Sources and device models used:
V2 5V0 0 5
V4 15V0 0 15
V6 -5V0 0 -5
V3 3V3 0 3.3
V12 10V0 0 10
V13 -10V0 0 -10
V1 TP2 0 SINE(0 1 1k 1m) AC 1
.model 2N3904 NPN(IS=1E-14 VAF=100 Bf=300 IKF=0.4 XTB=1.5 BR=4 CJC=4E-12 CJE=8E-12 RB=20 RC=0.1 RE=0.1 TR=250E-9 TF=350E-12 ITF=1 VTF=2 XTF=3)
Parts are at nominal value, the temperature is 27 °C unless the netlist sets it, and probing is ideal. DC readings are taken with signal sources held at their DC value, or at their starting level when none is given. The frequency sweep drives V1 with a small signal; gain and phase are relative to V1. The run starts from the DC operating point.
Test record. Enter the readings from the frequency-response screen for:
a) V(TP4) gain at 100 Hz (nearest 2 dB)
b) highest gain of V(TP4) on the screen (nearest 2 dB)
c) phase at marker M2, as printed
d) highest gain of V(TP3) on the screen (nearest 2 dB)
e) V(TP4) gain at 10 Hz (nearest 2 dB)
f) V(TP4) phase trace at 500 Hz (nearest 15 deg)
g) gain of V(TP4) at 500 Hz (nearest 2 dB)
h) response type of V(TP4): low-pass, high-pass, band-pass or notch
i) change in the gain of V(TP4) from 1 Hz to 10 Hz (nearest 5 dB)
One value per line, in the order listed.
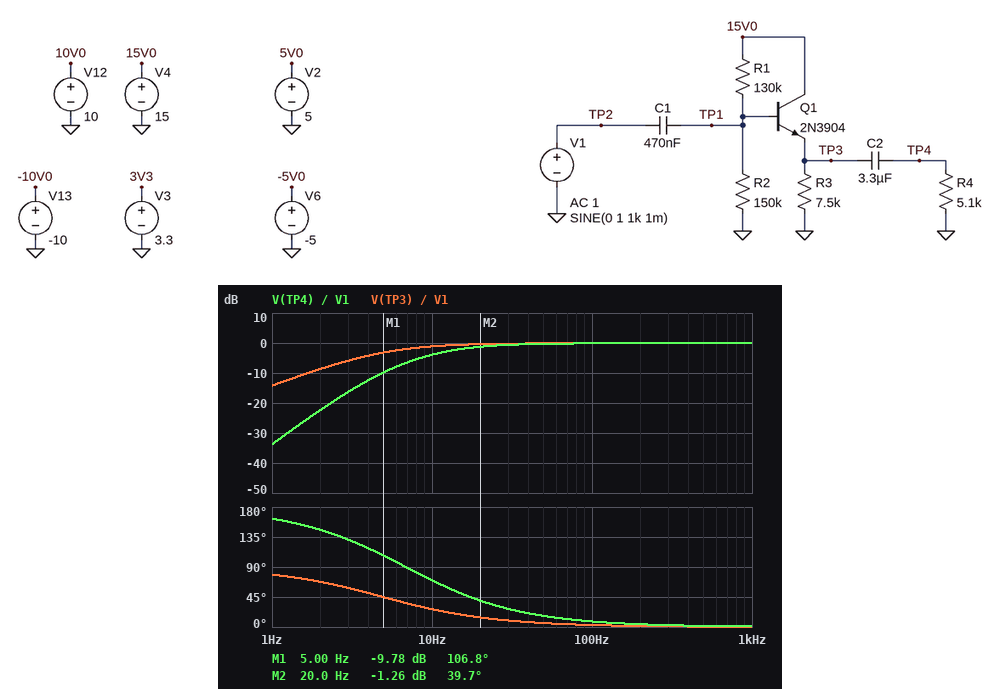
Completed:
0 dB
0 dB
39.7 deg
0 dB
-4 dB
0 deg
0 dB
high-pass
30 dB
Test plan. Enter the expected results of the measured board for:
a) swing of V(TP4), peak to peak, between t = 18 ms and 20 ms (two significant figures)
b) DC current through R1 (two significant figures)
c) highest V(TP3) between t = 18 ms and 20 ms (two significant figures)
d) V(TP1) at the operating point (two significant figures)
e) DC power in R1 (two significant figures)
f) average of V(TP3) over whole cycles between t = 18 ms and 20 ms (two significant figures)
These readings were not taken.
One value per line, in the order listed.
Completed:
2.0 V
55 µA
8.2 V
7.8 V
400 µW
7.2 V
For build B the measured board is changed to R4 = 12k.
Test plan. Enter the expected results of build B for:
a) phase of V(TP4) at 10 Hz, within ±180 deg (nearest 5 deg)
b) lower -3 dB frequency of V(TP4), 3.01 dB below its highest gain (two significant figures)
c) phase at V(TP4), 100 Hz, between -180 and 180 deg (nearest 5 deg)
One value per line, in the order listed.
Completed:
50 deg
7.1 Hz
5 deg
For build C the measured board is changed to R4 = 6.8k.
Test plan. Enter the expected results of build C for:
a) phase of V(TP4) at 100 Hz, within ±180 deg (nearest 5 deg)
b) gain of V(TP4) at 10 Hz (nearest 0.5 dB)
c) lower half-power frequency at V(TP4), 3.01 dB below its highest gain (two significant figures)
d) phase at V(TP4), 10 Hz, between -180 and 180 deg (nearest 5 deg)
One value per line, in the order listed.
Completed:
5 deg
-3.0 dB
9.6 Hz
60 deg
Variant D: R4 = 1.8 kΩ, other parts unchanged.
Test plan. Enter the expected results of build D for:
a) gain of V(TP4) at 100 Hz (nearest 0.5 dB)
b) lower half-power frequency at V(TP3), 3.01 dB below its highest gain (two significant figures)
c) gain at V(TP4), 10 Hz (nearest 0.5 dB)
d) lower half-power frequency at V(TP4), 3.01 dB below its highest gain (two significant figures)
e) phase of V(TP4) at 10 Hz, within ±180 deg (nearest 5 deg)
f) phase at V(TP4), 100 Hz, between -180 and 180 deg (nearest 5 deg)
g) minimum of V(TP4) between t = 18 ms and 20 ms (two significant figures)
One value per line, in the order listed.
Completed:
-0.5 dB
5.0 Hz
-10.5 dB
28 Hz
95 deg
20 deg
-970 mV
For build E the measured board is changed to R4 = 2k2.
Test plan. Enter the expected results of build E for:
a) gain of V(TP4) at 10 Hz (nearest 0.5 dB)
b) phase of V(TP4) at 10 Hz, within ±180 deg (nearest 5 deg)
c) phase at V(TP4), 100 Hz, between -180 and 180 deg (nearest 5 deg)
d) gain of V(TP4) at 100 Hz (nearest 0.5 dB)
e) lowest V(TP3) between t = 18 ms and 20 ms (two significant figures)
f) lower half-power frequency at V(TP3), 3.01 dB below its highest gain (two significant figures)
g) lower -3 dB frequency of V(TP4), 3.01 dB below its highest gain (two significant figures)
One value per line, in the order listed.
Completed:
-9.0 dB
90 deg
15 deg
-0.5 dB
6.2 V
5.0 Hz
23 Hz
